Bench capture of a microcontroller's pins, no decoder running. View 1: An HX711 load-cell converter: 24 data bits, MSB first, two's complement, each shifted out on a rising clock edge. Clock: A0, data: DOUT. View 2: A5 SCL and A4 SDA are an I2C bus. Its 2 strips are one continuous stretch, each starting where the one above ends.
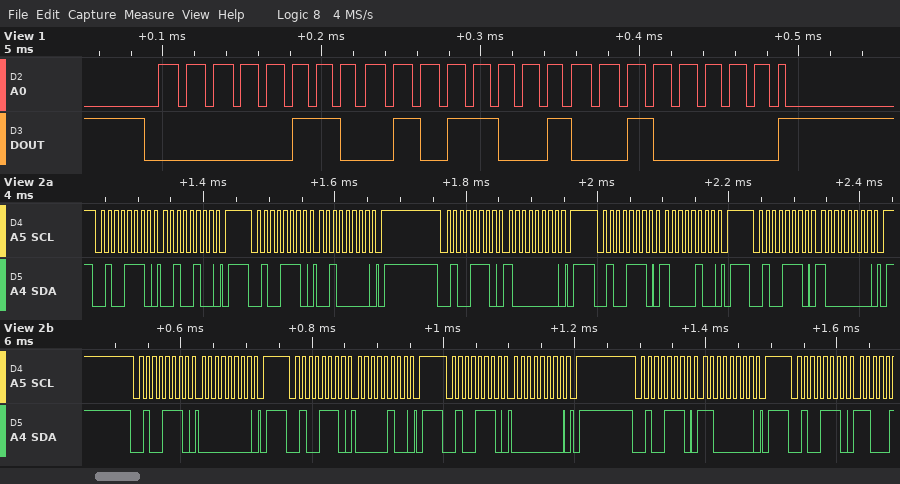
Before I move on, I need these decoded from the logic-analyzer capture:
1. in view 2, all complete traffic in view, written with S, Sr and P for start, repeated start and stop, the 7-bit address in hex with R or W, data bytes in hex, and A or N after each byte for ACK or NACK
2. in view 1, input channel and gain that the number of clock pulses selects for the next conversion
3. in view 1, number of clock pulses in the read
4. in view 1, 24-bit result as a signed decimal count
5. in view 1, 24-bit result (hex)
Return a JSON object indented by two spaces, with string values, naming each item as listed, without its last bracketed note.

{
  "in view 2, all complete traffic in view, written with S, Sr and P for start, repeated start and stop, the 7-bit address in hex with R or W, data bytes in hex, and A or N after each byte for ACK or NACK": "S 27W A 24 A P S 27W A 20 A P S 27W A 80 A P S 27W A 84 A P S 27W A 80 A P S 27W A 00 A P S 27W A 04 A P S 27W A 00 A P S 27W A C0 A P S 27W A",
  "in view 1, input channel and gain that the number of clock pulses selects for the next conversion": "channel A, gain 128",
  "in view 1, number of clock pulses in the read": "25",
  "in view 1, 24-bit result as a signed decimal count": "416032",
  "in view 1, 24-bit result": "0x065920"
}
